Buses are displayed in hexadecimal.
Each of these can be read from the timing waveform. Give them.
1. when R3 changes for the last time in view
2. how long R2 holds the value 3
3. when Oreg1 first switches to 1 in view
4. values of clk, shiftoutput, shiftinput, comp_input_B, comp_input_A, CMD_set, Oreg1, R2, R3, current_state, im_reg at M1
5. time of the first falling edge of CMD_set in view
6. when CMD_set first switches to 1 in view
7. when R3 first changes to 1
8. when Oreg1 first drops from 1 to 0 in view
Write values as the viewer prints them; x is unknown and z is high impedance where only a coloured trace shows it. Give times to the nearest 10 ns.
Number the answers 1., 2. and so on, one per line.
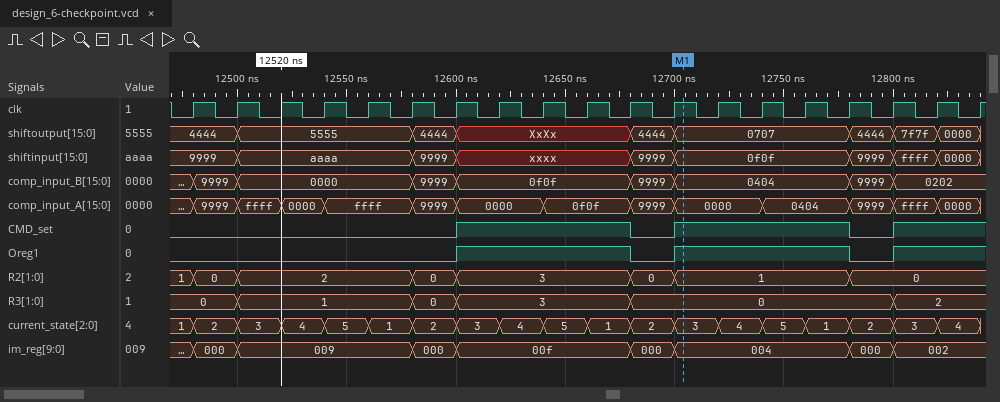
1. 12800 ns
2. 80 ns
3. 12600 ns
4. clk=1, shiftoutput=0707, shiftinput=0f0f, comp_input_B=0404, comp_input_A=0000, CMD_set=1, Oreg1=1, R2=1, R3=0, current_state=3, im_reg=004
5. 12680 ns
6. 12600 ns
7. 12500 ns
8. 12680 ns
